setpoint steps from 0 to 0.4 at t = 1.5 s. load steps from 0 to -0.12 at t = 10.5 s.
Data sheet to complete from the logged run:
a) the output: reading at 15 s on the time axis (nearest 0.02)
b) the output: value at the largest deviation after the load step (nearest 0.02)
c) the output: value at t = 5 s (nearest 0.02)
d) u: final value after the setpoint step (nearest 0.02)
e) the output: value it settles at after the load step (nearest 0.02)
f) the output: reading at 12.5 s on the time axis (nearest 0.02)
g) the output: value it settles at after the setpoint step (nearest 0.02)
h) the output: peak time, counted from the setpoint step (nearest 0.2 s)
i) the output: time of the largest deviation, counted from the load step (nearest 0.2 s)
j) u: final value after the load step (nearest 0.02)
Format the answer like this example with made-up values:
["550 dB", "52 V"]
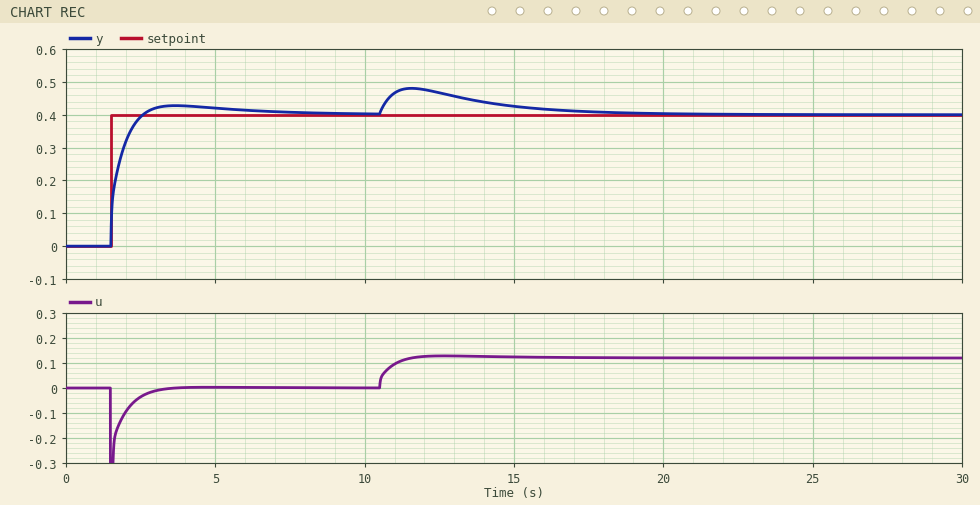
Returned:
["0.42", "0.48", "0.42", "0.00", "0.40", "0.46", "0.40", "2.2 s", "1.0 s", "0.12"]
